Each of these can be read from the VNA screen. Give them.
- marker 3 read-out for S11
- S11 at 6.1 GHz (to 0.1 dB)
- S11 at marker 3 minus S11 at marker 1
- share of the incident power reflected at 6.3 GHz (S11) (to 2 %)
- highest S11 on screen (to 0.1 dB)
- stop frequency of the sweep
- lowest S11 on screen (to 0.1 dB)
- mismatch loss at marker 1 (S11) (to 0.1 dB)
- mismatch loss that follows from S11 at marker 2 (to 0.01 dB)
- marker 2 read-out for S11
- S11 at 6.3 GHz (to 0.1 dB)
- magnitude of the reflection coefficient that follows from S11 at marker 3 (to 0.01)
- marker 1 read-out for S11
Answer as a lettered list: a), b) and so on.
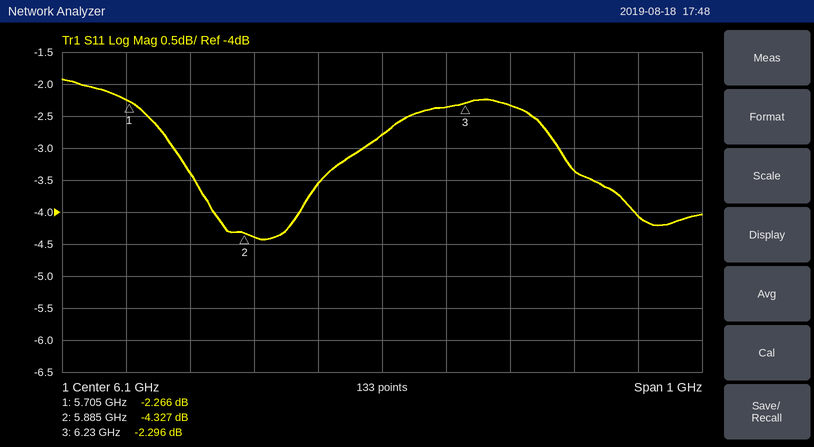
a) -2.296 dB
b) -2.8 dB
c) -0.030 dB
d) 58 %
e) -1.9 dB
f) 6.6 GHz
g) -4.4 dB
h) 3.9 dB
i) 2.00 dB
j) -4.327 dB
k) -2.3 dB
l) 0.77
m) -2.266 dB
